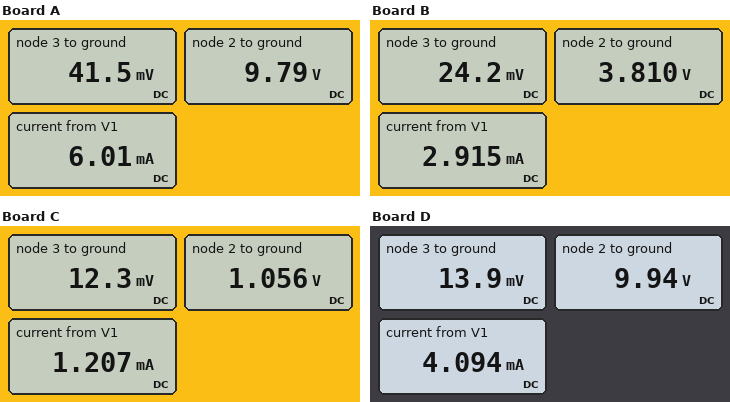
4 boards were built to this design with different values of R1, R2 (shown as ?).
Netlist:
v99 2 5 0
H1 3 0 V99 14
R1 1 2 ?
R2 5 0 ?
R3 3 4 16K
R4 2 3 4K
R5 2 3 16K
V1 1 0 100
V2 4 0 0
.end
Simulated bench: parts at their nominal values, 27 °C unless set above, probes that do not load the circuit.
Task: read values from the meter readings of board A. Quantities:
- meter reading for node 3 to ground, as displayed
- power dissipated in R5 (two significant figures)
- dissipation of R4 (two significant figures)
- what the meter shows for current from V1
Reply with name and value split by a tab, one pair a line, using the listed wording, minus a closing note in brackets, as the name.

meter reading for node 3 to ground, as displayed	41.5 mV
power dissipated in R5	5.9 mW
dissipation of R4	24 mW
what the meter shows for current from V1	6.01 mA
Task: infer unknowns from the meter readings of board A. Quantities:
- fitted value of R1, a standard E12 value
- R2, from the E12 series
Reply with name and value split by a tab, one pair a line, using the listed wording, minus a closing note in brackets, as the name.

fitted value of R1, a standard E12 value	15 kΩ
R2, from the E12 series	3.3 kΩ
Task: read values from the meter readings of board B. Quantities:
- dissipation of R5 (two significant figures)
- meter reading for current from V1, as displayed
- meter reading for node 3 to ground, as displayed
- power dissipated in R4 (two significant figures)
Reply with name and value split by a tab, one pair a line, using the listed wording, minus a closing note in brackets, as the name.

dissipation of R5	900 µW
meter reading for current from V1, as displayed	2.915 mA
meter reading for node 3 to ground, as displayed	24.2 mV
power dissipated in R4	3.6 mW
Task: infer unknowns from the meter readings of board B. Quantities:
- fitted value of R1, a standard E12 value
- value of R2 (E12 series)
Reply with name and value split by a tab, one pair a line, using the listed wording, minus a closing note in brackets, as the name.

fitted value of R1, a standard E12 value	33 kΩ
value of R2	2.2 kΩ
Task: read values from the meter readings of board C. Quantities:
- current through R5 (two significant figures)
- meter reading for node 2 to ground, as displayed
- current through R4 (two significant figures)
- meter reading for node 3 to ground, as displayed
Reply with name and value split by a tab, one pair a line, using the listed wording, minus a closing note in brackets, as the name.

current through R5	65 µA
meter reading for node 2 to ground, as displayed	1.056 V
current through R4	260 µA
meter reading for node 3 to ground, as displayed	12.3 mV
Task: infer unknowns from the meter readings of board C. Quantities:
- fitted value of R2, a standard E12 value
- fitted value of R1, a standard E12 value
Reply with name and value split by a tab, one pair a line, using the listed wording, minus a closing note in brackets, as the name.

fitted value of R2, a standard E12 value	1.2 kΩ
fitted value of R1, a standard E12 value	82 kΩ
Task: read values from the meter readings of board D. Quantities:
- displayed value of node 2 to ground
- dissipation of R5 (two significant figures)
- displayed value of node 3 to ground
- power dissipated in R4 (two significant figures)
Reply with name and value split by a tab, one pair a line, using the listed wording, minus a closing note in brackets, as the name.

displayed value of node 2 to ground	9.94 V
dissipation of R5	6.2 mW
displayed value of node 3 to ground	13.9 mV
power dissipated in R4	25 mW
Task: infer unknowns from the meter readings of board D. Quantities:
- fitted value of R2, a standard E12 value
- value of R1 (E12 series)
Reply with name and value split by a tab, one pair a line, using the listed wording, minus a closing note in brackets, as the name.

fitted value of R2, a standard E12 value	10 kΩ
value of R1	22 kΩ
